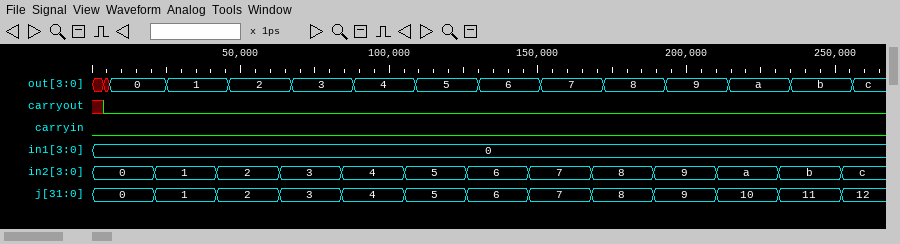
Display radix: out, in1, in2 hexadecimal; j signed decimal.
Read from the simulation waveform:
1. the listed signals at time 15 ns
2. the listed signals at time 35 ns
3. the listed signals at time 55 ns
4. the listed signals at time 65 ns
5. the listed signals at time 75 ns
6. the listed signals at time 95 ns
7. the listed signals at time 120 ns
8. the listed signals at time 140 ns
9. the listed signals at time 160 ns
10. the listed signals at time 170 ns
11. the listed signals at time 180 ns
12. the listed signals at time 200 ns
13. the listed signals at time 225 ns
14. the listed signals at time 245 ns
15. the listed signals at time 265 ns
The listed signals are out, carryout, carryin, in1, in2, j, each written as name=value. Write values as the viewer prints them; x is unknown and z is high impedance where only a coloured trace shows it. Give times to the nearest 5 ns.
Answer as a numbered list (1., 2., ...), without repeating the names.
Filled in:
1. out=0, carryout=0, carryin=0, in1=0, in2=0, j=0
2. out=1, carryout=0, carryin=0, in1=0, in2=1, j=1
3. out=2, carryout=0, carryin=0, in1=0, in2=2, j=2
4. out=2, carryout=0, carryin=0, in1=0, in2=3, j=3
5. out=3, carryout=0, carryin=0, in1=0, in2=3, j=3
6. out=4, carryout=0, carryin=0, in1=0, in2=4, j=4
7. out=5, carryout=0, carryin=0, in1=0, in2=5, j=5
8. out=6, carryout=0, carryin=0, in1=0, in2=6, j=6
9. out=7, carryout=0, carryin=0, in1=0, in2=7, j=7
10. out=7, carryout=0, carryin=0, in1=0, in2=8, j=8
11. out=8, carryout=0, carryin=0, in1=0, in2=8, j=8
12. out=9, carryout=0, carryin=0, in1=0, in2=9, j=9
13. out=a, carryout=0, carryin=0, in1=0, in2=a, j=10
14. out=b, carryout=0, carryin=0, in1=0, in2=b, j=11
15. out=c, carryout=0, carryin=0, in1=0, in2=c, j=12
